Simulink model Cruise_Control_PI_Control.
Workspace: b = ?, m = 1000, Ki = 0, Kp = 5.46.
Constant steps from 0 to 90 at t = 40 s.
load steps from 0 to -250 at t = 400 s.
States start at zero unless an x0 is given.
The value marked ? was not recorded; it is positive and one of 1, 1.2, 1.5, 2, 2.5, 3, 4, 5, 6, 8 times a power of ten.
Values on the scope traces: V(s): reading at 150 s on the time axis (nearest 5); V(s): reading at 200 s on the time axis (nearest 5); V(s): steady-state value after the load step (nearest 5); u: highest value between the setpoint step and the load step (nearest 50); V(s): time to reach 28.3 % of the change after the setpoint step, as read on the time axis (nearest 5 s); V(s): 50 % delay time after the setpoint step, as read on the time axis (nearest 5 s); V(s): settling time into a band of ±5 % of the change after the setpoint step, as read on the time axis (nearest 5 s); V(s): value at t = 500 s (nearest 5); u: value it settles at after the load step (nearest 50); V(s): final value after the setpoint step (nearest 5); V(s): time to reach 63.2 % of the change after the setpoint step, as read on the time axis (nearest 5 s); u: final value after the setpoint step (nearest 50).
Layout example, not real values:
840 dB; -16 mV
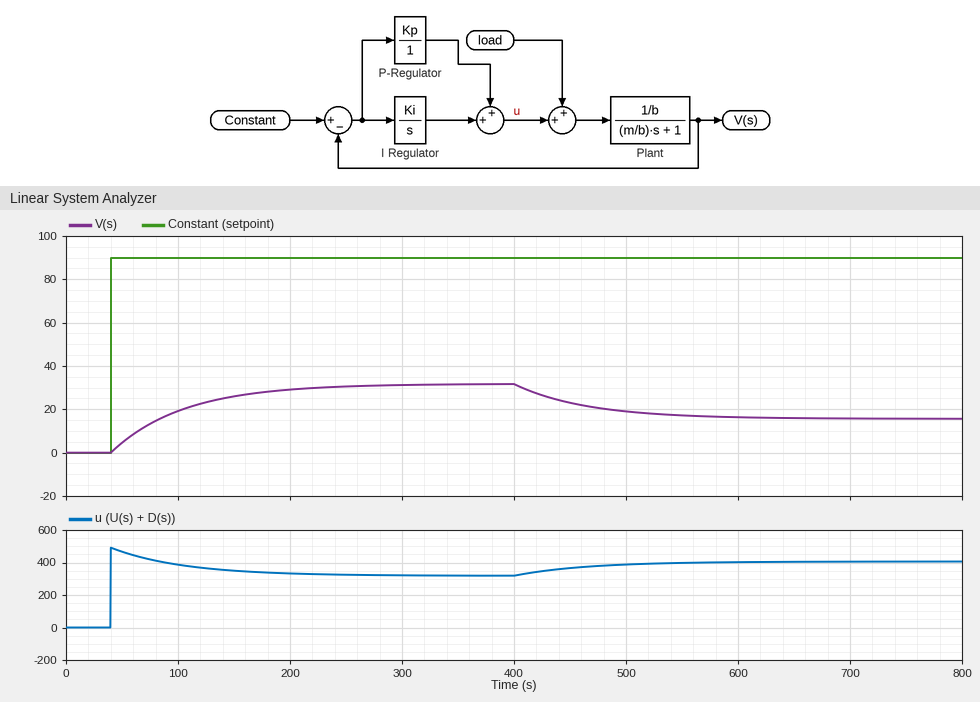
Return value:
25; 30; 15; 500; 60 s; 85 s; 235 s; 20; 400; 30; 105 s; 300
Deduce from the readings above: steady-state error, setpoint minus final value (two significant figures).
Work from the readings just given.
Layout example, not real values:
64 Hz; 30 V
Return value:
60
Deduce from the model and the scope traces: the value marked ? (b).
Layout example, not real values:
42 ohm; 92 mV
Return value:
10
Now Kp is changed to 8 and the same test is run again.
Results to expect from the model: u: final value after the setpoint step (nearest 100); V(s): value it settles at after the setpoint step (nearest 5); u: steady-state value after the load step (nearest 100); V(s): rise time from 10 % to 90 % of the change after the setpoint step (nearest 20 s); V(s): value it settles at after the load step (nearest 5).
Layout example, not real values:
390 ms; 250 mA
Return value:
400; 40; 500; 120 s; 25
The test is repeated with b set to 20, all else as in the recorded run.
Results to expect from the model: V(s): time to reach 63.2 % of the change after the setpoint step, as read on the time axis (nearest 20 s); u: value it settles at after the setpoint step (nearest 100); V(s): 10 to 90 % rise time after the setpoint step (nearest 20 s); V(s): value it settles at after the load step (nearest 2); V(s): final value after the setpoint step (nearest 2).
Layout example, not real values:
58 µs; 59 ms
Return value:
80 s; 400; 80 s; 10; 20
